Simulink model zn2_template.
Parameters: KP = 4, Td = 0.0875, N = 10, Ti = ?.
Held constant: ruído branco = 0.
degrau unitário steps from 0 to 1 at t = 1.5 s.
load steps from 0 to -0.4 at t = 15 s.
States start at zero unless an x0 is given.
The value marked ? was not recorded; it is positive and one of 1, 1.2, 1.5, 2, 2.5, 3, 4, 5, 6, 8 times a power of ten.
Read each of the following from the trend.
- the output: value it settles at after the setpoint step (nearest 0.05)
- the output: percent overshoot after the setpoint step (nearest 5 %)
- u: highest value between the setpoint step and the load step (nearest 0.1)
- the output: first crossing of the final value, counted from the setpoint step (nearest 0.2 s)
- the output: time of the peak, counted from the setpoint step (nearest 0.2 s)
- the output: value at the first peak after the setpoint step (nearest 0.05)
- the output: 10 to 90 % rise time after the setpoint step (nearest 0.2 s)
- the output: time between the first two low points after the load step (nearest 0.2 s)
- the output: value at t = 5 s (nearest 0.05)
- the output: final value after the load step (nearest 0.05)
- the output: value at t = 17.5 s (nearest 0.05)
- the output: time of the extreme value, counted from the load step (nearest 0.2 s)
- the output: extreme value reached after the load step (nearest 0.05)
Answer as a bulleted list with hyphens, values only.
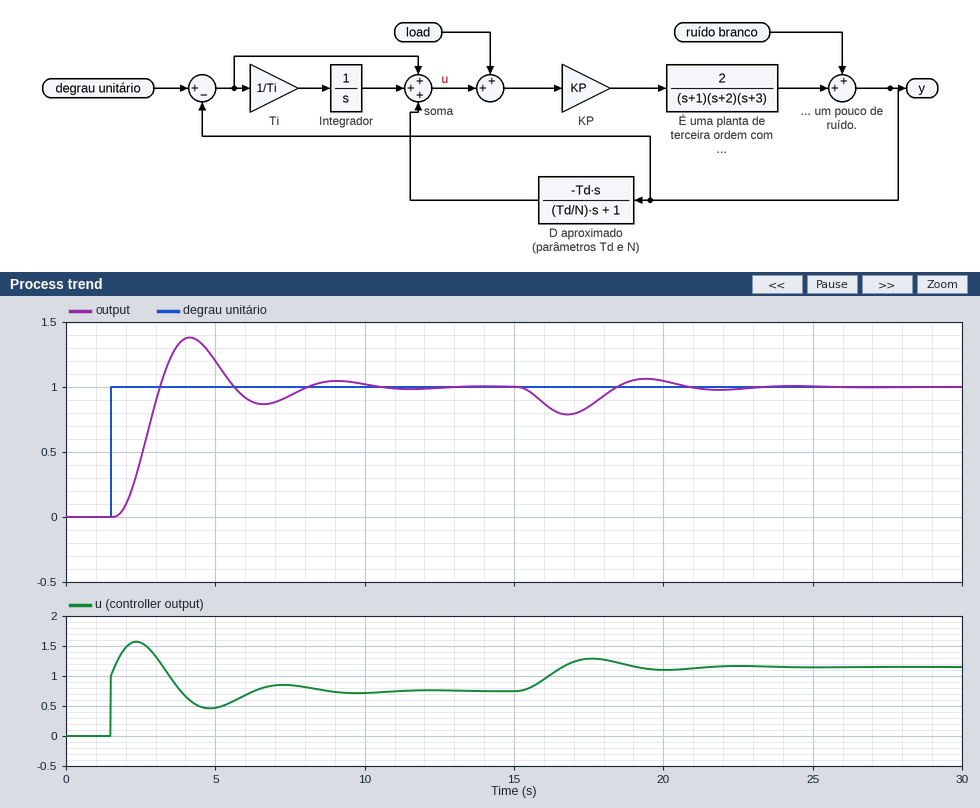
- 1.00
- 40 %
- 1.6
- 1.6 s
- 2.6 s
- 1.40
- 1.0 s
- 5.0 s
- 1.20
- 1.00
- 0.85
- 1.8 s
- 0.80
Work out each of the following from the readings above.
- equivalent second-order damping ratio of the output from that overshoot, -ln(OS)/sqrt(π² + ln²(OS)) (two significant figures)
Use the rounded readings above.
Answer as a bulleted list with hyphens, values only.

- 0.28
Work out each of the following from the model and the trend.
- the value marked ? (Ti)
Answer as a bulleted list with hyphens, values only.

- 0.8
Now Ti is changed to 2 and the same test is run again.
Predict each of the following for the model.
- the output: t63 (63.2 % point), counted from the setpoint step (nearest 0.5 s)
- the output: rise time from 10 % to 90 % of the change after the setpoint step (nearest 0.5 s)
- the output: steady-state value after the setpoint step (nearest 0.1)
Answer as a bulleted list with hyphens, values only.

- 1.5 s
- 1.5 s
- 1.0
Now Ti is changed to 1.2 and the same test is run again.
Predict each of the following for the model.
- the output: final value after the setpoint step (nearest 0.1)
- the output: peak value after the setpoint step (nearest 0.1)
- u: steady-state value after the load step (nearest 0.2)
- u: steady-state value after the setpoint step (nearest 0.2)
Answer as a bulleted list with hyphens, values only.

- 1.0
- 1.2
- 1.2
- 0.8
